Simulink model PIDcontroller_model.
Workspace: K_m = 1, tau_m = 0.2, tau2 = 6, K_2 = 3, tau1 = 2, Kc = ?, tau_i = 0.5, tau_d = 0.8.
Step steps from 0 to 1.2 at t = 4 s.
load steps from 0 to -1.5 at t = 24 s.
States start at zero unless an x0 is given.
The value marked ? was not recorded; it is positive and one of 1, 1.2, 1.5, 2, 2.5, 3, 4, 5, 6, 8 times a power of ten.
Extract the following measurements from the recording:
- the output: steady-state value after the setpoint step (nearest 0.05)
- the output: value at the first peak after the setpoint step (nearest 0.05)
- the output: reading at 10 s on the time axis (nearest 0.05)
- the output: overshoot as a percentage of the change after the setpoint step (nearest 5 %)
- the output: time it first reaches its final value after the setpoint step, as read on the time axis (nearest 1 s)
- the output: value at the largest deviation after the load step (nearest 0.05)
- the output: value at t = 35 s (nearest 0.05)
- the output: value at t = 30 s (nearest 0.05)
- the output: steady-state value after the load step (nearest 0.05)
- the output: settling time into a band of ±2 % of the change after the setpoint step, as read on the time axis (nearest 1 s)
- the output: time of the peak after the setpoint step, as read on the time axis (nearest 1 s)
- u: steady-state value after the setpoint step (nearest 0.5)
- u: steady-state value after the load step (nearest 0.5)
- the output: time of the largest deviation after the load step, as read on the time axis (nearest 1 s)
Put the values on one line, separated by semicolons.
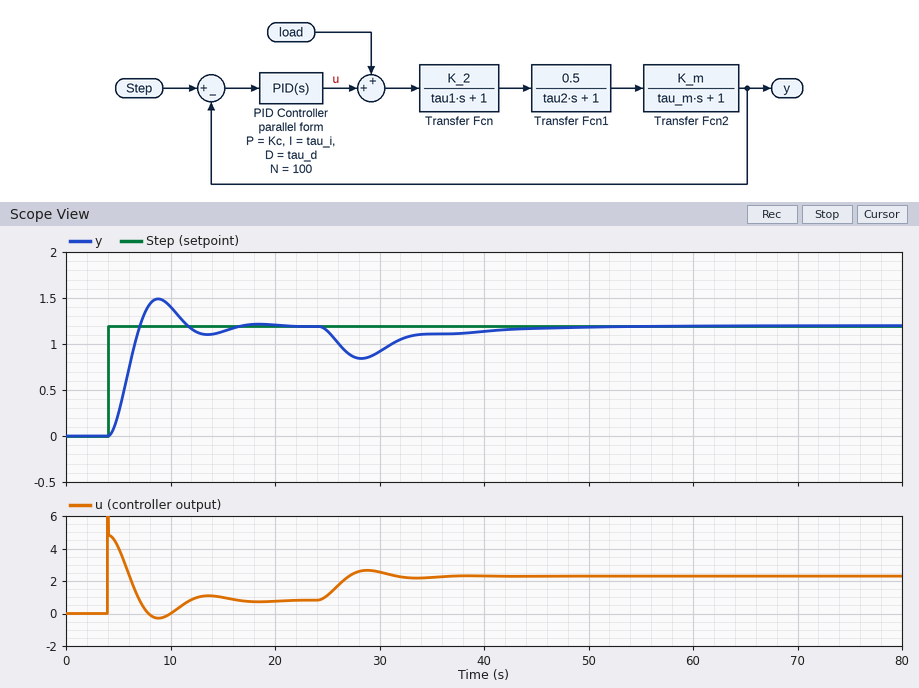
1.20; 1.50; 1.40; 25 %; 7 s; 0.85; 1.10; 0.90; 1.20; 16 s; 9 s; 1.0; 2.5; 28 s
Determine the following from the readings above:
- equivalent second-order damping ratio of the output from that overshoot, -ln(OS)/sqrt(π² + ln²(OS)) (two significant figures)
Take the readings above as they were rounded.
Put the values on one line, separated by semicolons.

0.40
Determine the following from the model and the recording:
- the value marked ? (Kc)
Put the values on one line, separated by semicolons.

4
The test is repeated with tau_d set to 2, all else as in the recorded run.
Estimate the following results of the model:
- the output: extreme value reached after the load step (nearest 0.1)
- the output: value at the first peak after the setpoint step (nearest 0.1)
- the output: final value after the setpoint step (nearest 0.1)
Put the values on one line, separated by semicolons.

0.9; 1.4; 1.2
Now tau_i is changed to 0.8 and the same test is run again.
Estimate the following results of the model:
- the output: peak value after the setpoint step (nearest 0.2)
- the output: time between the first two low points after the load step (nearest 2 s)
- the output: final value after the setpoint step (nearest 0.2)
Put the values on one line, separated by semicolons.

1.6; 10 s; 1.2
